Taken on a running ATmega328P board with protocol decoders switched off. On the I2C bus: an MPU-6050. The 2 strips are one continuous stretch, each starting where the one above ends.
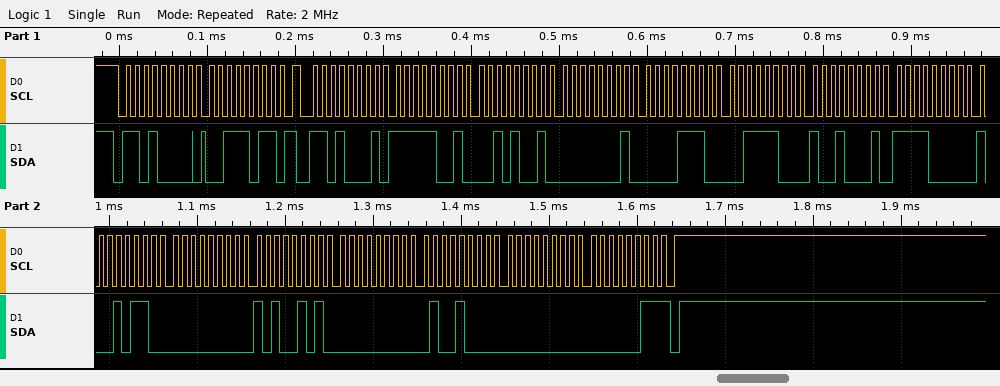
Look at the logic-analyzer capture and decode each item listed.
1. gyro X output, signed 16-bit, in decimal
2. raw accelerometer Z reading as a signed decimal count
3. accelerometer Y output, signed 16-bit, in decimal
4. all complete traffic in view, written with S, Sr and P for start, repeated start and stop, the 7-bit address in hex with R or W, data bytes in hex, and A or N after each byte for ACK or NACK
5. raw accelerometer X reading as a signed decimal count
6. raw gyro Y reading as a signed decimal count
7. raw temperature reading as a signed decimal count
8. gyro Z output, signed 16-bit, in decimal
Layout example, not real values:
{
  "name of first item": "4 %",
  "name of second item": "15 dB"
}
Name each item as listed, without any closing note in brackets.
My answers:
{
  "gyro X output, signed 16-bit, in decimal": "165",
  "raw accelerometer Z reading as a signed decimal count": "15505",
  "accelerometer Y output, signed 16-bit, in decimal": "270",
  "all complete traffic in view, written with S, Sr and P for start, repeated start and stop, the 7-bit address in hex with R or W, data bytes in hex, and A or N after each byte for ACK or NACK": "S 68W A 3B A Sr 68R A F9 A 29 A 01 A 0E A 3C A 91 A F0 A 96 A 00 A A5 A 00 A 48 A 00 A 03 N P",
  "raw accelerometer X reading as a signed decimal count": "-1751",
  "raw gyro Y reading as a signed decimal count": "72",
  "raw temperature reading as a signed decimal count": "-3946",
  "gyro Z output, signed 16-bit, in decimal": "3"
}
